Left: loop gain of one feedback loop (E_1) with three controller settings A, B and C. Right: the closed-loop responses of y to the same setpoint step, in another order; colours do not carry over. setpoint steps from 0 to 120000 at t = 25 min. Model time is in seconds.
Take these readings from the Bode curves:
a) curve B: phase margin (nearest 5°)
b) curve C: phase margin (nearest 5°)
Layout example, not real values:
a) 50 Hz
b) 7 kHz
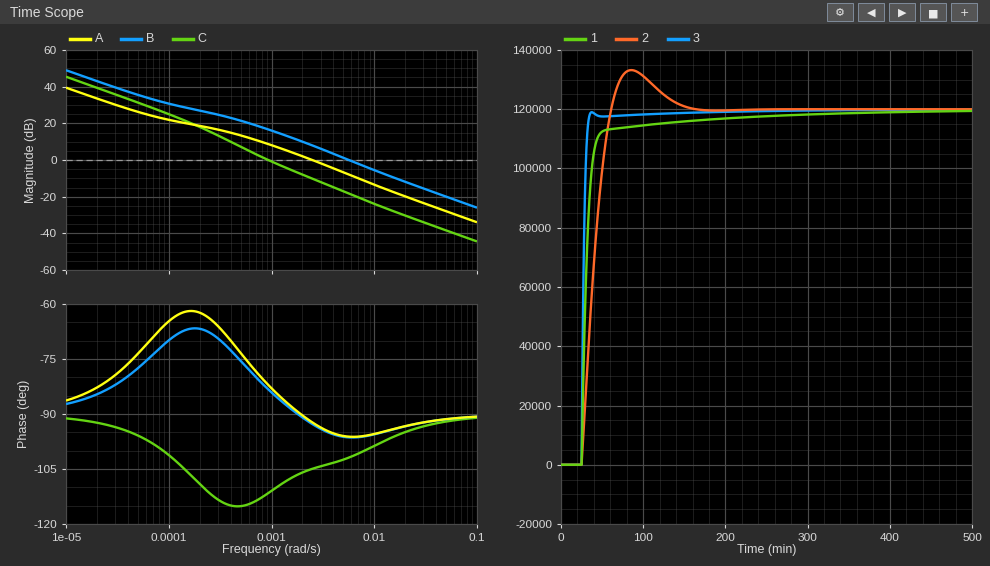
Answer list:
a) 85°
b) 70°
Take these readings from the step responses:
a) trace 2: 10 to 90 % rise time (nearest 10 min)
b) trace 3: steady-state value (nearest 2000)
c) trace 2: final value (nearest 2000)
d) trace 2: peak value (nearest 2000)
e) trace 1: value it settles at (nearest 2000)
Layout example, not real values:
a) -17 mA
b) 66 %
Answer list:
a) 30 min
b) 120000
c) 120000
d) 134000
e) 120000
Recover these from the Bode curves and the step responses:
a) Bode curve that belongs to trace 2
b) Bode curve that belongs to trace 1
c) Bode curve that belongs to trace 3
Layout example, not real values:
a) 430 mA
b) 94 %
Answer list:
a) C
b) A
c) B
